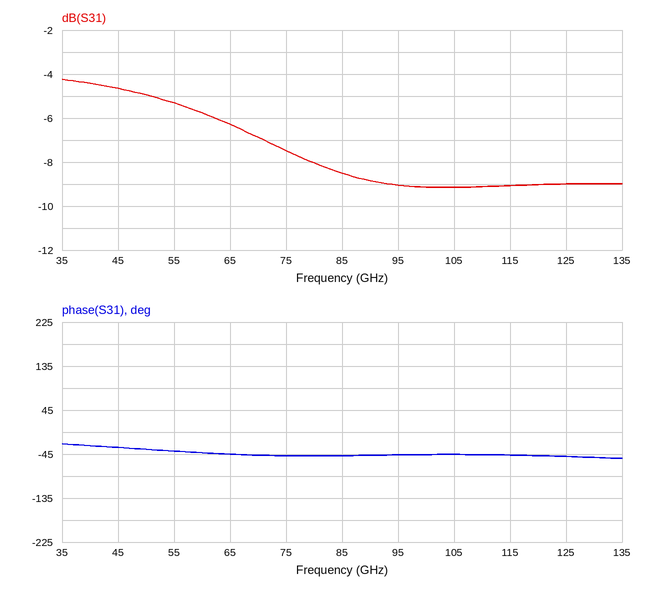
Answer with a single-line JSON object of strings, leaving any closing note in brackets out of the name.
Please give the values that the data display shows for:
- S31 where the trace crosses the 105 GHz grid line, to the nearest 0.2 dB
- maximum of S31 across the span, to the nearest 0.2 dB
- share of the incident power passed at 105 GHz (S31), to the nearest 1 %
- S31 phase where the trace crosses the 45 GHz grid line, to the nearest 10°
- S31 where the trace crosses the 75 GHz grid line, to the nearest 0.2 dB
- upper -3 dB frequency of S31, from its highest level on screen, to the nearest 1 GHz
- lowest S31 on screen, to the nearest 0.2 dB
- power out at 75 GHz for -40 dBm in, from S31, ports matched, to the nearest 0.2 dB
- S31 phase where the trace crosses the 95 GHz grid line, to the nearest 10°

{"S31 where the trace crosses the 105 GHz grid line, to the nearest 0.2 dB": "-9.2 dB", "maximum of S31 across the span, to the nearest 0.2 dB": "-4.2 dB", "share of the incident power passed at 105 GHz (S31), to the nearest 1 %": "12 %", "S31 phase where the trace crosses the 45 GHz grid line, to the nearest 10°": "-30°", "S31 where the trace crosses the 75 GHz grid line, to the nearest 0.2 dB": "-7.4 dB", "upper -3 dB frequency of S31, from its highest level on screen, to the nearest 1 GHz": "73 GHz", "lowest S31 on screen, to the nearest 0.2 dB": "-9.2 dB", "power out at 75 GHz for -40 dBm in, from S31, ports matched, to the nearest 0.2 dB": "-47.4 dBm", "S31 phase where the trace crosses the 95 GHz grid line, to the nearest 10°": "-50°"}
